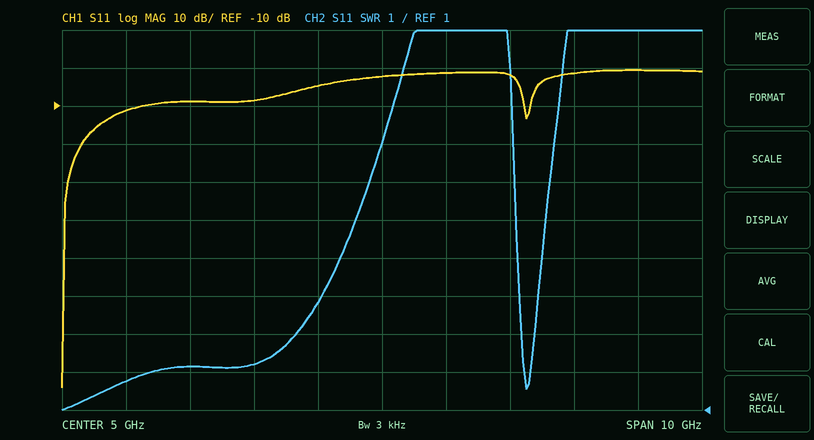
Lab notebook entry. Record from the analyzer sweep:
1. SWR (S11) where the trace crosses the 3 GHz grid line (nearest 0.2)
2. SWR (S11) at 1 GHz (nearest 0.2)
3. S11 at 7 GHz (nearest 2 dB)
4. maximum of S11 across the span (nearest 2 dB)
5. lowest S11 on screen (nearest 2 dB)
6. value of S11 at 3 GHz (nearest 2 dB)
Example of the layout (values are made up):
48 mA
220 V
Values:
2.2
1.8
-2 dB
0 dB
-84 dB
-8 dB
